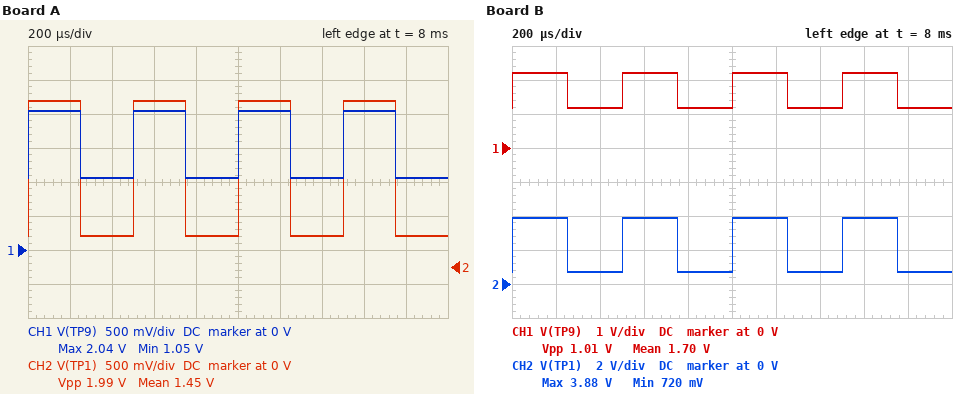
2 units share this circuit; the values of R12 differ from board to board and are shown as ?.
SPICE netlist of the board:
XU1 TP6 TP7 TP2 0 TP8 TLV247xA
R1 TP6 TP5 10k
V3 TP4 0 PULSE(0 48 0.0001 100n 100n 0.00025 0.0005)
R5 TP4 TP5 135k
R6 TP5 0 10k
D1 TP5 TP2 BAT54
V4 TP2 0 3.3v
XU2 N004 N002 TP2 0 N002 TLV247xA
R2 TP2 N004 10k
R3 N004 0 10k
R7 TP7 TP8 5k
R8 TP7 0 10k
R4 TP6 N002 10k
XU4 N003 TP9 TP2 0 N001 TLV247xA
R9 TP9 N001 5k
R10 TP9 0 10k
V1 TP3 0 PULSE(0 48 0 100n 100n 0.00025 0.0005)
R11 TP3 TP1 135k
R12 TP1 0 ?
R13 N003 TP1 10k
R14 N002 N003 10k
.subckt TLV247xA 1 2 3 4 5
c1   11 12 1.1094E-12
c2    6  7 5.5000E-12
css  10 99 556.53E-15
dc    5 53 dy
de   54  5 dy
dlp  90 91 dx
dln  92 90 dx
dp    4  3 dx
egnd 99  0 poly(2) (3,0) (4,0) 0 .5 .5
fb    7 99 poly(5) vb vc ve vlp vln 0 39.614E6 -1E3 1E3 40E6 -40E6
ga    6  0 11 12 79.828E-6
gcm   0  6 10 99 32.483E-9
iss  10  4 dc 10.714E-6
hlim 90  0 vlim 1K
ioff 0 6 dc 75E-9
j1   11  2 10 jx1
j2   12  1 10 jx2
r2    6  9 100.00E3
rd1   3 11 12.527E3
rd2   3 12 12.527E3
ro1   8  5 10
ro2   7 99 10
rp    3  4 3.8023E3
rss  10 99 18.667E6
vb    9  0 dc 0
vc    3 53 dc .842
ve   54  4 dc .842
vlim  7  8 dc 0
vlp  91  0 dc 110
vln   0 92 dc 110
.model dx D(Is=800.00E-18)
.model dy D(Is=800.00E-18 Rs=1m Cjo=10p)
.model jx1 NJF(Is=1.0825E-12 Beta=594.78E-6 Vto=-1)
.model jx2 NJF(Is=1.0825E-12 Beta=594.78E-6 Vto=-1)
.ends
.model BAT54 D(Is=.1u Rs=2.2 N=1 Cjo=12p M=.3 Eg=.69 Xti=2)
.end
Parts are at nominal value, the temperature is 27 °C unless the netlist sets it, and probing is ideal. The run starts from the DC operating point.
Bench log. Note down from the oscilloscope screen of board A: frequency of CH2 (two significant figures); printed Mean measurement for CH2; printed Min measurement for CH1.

2.0 kHz
1.45 V
1.05 V
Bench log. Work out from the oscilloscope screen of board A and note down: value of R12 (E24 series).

8.2 kΩ
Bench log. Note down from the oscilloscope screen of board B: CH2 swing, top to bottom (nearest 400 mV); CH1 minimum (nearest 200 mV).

3.2 V
1.2 V
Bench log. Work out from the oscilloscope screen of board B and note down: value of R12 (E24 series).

18 kΩ
